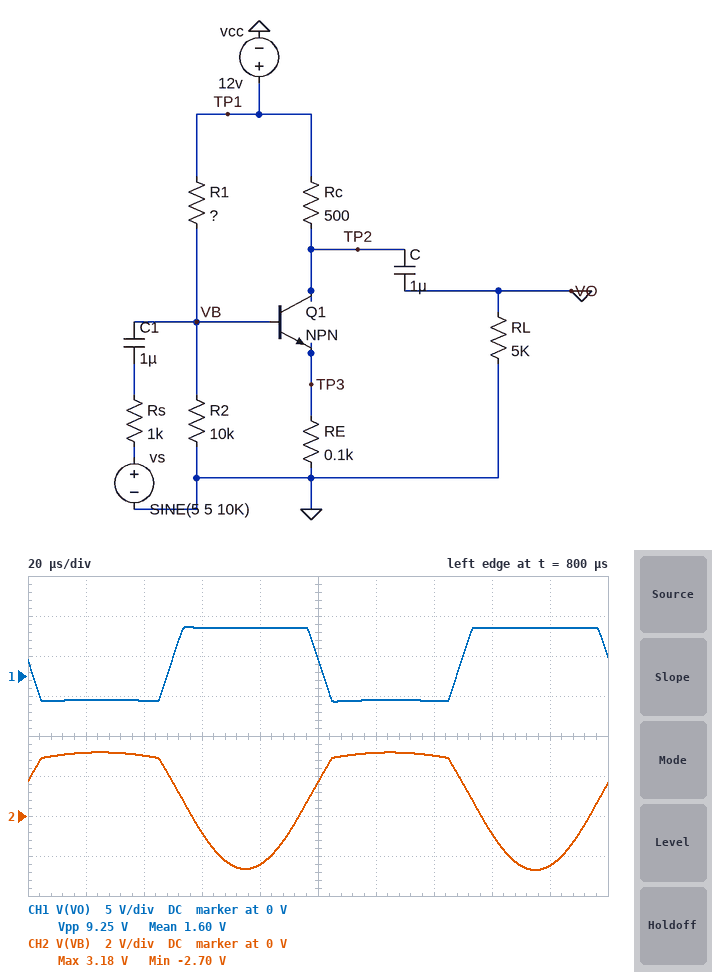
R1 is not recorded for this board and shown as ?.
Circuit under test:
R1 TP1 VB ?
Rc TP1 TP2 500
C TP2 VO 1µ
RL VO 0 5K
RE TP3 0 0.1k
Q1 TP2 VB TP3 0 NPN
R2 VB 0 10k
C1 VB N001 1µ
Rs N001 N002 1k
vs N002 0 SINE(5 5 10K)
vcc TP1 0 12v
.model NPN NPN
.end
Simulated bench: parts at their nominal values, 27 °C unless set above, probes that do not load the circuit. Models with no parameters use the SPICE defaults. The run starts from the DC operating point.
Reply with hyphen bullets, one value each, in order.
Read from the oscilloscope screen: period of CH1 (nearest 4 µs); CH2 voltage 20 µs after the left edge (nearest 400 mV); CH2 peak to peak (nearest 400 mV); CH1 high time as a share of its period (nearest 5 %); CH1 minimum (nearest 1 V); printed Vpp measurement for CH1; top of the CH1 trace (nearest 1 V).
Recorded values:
- 100 µs
- 3.2 V
- 6.0 V
- 50 %
- -3 V
- 9.25 V
- 6 V
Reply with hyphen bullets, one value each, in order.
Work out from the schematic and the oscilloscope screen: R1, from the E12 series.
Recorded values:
- 27 kΩ
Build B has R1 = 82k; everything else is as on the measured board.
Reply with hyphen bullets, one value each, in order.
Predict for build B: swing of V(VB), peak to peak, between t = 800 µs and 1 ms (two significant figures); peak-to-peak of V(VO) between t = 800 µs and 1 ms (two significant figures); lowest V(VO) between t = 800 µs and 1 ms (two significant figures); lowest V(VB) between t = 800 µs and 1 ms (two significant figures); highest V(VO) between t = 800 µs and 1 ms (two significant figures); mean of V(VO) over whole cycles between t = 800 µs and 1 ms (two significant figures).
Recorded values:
- 7.0 V
- 9.7 V
- -8.0 V
- -3.8 V
- 1.7 V
- -2.2 V
